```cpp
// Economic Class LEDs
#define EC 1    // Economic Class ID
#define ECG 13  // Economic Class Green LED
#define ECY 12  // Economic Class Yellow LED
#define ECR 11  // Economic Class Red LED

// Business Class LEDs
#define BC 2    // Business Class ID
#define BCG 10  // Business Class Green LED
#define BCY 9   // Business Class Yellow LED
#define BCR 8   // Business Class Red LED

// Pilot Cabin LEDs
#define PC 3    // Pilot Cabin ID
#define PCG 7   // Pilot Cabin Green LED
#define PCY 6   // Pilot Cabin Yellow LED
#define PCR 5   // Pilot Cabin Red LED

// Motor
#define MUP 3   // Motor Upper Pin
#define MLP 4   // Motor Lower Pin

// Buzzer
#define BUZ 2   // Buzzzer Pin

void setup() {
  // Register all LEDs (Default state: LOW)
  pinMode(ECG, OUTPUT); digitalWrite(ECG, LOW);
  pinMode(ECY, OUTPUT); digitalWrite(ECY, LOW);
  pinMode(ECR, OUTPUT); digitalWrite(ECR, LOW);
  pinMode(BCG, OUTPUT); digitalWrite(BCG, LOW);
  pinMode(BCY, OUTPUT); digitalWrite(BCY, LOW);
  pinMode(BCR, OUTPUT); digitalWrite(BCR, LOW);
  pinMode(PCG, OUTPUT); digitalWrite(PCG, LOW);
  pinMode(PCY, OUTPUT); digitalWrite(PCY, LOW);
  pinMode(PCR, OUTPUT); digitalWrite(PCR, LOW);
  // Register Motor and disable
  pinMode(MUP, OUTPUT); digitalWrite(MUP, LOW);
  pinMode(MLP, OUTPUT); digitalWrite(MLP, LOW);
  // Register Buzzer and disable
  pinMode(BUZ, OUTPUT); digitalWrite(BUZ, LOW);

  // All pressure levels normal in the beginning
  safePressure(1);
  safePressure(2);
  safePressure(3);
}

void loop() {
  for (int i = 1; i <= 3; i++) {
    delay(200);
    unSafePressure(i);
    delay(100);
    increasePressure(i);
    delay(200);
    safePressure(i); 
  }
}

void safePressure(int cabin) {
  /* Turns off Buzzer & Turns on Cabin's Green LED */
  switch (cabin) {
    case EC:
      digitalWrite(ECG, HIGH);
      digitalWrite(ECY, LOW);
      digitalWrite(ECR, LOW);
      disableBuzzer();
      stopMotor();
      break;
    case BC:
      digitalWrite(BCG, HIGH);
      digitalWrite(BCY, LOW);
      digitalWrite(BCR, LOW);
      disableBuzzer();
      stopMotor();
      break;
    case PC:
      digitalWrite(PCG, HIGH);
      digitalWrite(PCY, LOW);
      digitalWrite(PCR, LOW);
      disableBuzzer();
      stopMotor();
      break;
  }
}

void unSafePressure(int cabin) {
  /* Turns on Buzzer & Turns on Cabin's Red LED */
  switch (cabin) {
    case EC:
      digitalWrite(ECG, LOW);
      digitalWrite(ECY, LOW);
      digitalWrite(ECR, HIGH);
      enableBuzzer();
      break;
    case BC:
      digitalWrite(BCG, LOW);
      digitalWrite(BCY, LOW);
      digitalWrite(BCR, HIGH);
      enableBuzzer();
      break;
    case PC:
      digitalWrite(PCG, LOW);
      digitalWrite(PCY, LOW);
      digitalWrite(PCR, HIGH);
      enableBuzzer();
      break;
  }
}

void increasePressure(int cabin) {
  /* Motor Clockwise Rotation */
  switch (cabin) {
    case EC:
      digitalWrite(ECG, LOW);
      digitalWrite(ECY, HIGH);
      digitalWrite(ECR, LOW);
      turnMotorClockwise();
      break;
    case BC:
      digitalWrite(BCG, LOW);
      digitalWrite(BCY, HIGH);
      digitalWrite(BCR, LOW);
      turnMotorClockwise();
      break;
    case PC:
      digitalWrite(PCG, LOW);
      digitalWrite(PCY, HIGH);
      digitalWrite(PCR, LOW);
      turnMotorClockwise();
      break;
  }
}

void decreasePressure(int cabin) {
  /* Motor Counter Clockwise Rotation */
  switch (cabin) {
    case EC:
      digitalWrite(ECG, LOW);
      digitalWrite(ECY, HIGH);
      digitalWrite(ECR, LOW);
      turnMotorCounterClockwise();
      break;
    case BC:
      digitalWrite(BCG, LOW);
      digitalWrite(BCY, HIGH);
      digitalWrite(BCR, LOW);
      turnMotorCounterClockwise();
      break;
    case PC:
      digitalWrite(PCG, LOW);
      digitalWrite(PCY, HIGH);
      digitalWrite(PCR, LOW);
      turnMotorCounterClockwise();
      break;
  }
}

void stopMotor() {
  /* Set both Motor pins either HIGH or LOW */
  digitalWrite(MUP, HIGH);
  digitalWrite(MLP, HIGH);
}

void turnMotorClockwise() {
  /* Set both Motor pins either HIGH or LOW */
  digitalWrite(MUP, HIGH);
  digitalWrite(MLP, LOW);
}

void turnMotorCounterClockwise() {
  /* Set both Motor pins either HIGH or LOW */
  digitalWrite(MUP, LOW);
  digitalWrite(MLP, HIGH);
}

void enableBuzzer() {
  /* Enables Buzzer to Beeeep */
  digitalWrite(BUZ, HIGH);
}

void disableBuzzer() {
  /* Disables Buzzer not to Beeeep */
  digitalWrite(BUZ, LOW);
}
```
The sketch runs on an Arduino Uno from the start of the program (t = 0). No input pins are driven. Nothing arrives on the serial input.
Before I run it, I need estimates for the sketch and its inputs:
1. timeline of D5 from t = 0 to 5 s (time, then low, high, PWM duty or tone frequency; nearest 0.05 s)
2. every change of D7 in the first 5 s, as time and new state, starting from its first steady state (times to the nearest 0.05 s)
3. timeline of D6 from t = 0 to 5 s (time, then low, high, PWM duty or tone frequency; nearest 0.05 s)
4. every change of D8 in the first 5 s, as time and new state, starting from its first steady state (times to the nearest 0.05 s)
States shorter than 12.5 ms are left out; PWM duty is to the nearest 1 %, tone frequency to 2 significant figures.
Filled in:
0 s low; 1.2 s high; 1.3 s low; 2.7 s high; 2.8 s low; 4.2 s high; 4.3 s low
0 s high; 1.2 s low; 1.5 s high; 2.7 s low; 3 s high; 4.2 s low; 4.5 s high
0 s low; 1.3 s high; 1.5 s low; 2.8 s high; 3 s low; 4.3 s high; 4.5 s low
0 s low; 0.7 s high; 0.8 s low; 2.2 s high; 2.3 s low; 3.7 s high; 3.8 s low
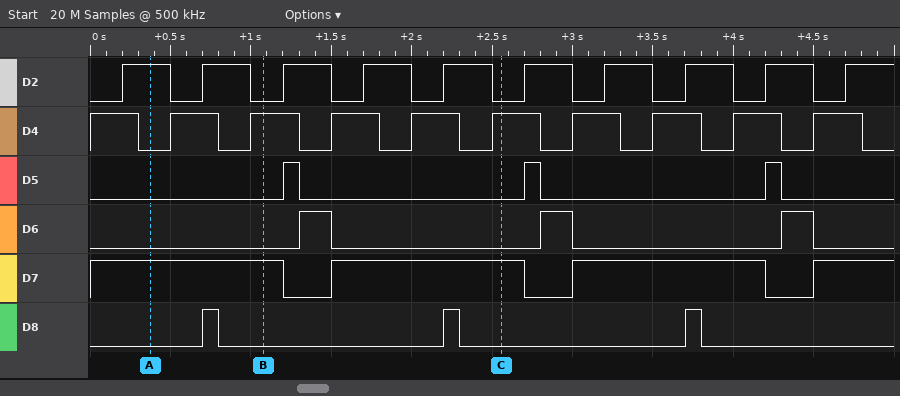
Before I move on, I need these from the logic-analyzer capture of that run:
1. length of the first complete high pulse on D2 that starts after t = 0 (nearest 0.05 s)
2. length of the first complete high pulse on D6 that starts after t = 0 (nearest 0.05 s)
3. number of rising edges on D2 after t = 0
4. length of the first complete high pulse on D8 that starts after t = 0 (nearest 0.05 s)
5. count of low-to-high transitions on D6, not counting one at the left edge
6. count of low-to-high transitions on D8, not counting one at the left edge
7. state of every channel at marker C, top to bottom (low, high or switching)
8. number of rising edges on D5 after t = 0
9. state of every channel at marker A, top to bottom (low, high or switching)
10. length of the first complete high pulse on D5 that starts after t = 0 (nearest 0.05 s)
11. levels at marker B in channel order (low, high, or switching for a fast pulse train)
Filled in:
0.30 s
0.20 s
10
0.10 s
3
3
D2 low, D4 high, D5 low, D6 low, D7 high, D8 low
3
D2 high, D4 low, D5 low, D6 low, D7 high, D8 low
0.10 s
D2 low, D4 high, D5 low, D6 low, D7 high, D8 low
